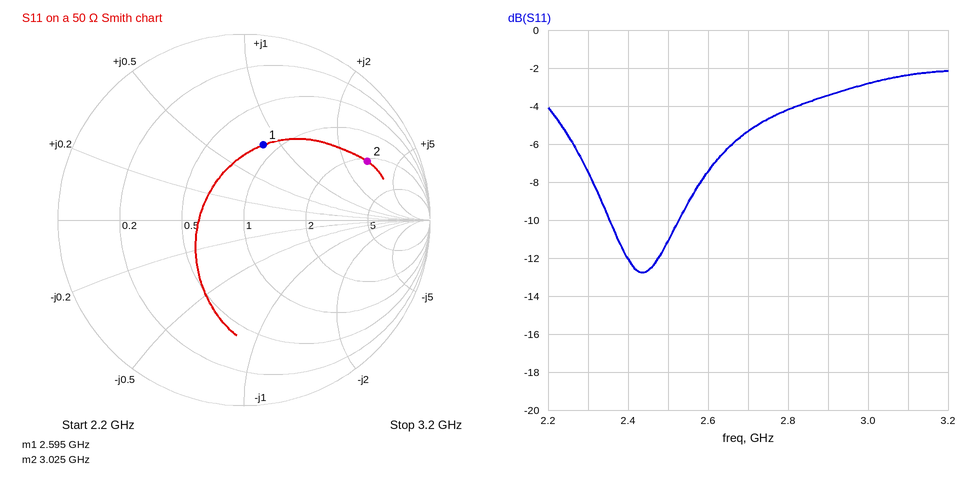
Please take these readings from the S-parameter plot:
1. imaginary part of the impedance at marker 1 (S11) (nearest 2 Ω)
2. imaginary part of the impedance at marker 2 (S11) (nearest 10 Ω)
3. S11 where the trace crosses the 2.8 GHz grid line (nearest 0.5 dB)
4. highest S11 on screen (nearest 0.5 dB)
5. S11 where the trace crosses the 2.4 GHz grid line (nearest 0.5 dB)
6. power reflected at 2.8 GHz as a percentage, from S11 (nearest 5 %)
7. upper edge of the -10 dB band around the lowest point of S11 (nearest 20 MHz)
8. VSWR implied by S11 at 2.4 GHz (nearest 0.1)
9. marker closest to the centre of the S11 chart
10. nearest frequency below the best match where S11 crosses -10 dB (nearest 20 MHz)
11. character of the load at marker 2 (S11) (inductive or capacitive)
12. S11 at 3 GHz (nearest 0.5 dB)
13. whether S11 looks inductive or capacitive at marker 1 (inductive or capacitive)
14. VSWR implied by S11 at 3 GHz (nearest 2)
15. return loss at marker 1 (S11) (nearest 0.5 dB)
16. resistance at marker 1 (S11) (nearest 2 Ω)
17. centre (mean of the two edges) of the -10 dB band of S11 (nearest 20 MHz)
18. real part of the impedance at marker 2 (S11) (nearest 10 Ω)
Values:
+42 Ω
+150 Ω
-4.0 dB
-2.0 dB
-12.0 dB
40 %
2.52 GHz
1.7
marker 1
2.36 GHz
inductive
-3.0 dB
inductive
6
7.5 dB
42 Ω
2.44 GHz
110 Ω
